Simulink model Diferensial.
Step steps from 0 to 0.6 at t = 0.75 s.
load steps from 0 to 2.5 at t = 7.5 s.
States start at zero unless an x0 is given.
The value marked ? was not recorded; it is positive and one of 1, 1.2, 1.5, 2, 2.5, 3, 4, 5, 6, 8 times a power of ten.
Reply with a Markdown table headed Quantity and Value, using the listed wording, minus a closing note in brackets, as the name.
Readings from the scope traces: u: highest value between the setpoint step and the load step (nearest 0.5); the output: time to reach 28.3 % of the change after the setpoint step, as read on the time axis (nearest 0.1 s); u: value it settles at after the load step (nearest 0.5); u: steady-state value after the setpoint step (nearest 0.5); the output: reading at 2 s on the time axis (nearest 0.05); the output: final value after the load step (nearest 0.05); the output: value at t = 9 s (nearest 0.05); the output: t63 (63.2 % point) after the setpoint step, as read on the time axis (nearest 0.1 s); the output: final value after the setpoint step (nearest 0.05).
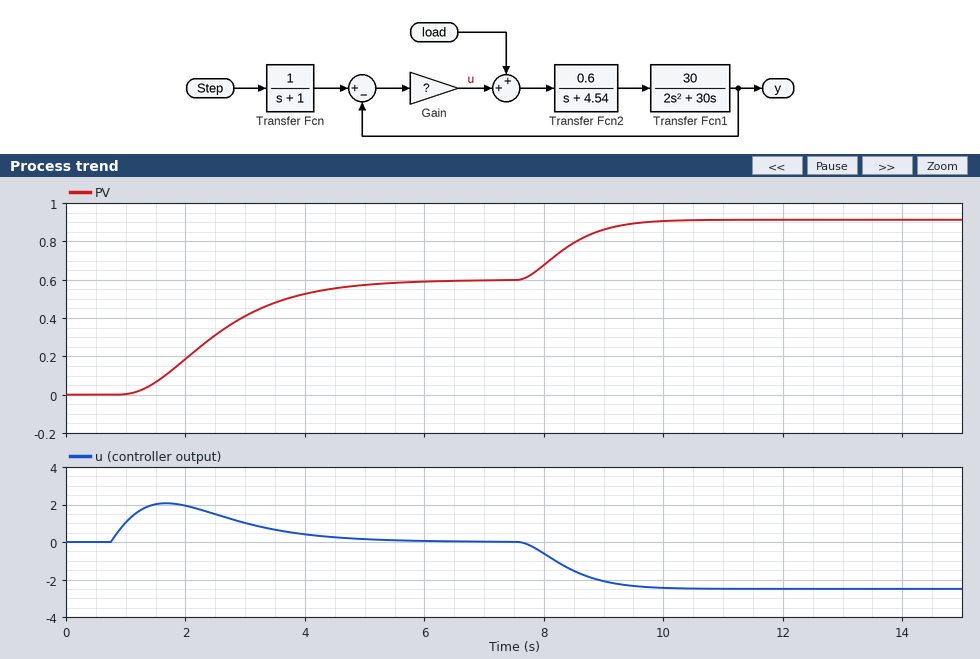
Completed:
| Quantity | Value |
|---|---|
| u: highest value between the setpoint step and the load step | 2.0 |
| the output: time to reach 28.3 % of the change after the setpoint step, as read on the time axis | 1.9 s |
| u: value it settles at after the load step | -2.5 |
| u: steady-state value after the setpoint step | 0.0 |
| the output: reading at 2 s on the time axis | 0.20 |
| the output: final value after the load step | 0.90 |
| the output: value at t = 9 s | 0.85 |
| the output: t63 (63.2 % point) after the setpoint step, as read on the time axis | 2.8 s |
| the output: final value after the setpoint step | 0.60 |
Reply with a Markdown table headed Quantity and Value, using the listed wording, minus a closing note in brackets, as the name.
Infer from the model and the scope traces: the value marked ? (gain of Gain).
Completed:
| Quantity | Value |
|---|---|
| the value marked ? | 8 |
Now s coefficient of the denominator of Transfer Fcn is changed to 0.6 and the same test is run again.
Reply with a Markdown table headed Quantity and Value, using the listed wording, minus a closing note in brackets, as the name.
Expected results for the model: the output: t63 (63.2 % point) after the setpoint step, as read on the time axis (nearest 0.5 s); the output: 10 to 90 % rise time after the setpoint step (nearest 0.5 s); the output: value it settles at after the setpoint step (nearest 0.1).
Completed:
| Quantity | Value |
|---|---|
| the output: t63 (63.2 % point) after the setpoint step, as read on the time axis | 2.5 s |
| the output: 10 to 90 % rise time after the setpoint step | 2.0 s |
| the output: value it settles at after the setpoint step | 0.6 |
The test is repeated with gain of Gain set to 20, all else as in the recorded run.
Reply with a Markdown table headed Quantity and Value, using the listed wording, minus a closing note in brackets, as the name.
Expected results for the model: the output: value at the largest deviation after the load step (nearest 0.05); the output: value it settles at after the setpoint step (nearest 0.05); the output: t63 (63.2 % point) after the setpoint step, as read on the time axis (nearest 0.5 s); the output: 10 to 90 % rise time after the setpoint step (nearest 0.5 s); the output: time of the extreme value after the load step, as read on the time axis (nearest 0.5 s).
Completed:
| Quantity | Value |
|---|---|
| the output: value at the largest deviation after the load step | 0.75 |
| the output: value it settles at after the setpoint step | 0.60 |
| the output: t63 (63.2 % point) after the setpoint step, as read on the time axis | 2.0 s |
| the output: 10 to 90 % rise time after the setpoint step | 2.0 s |
| the output: time of the extreme value after the load step, as read on the time axis | 8.5 s |
